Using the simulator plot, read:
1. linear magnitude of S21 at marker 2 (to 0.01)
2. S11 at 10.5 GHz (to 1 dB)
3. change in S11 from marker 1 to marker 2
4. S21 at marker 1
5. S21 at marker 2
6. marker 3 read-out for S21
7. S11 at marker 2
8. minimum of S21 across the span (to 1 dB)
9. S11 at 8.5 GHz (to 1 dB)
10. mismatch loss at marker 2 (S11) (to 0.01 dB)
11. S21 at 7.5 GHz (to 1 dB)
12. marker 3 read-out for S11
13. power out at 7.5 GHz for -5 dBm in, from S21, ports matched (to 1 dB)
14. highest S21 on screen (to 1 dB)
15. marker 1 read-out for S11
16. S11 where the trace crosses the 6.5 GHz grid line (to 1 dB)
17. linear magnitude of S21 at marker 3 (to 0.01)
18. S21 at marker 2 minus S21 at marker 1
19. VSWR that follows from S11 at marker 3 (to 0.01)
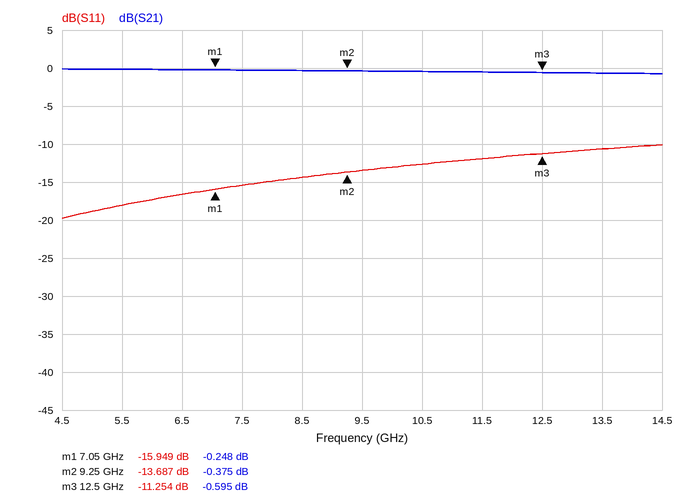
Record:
0.96
-13 dB
2.262 dB
-0.248 dB
-0.375 dB
-0.595 dB
-13.687 dB
-1 dB
-14 dB
0.19 dB
0 dB
-11.254 dB
-5 dBm
0 dB
-15.949 dB
-17 dB
0.93
-0.127 dB
1.75
